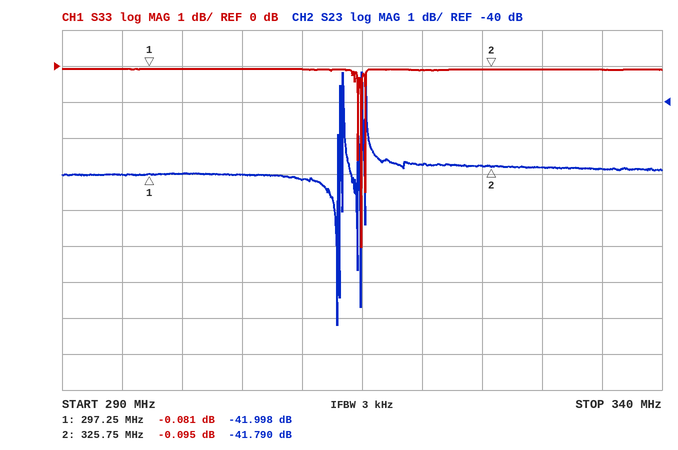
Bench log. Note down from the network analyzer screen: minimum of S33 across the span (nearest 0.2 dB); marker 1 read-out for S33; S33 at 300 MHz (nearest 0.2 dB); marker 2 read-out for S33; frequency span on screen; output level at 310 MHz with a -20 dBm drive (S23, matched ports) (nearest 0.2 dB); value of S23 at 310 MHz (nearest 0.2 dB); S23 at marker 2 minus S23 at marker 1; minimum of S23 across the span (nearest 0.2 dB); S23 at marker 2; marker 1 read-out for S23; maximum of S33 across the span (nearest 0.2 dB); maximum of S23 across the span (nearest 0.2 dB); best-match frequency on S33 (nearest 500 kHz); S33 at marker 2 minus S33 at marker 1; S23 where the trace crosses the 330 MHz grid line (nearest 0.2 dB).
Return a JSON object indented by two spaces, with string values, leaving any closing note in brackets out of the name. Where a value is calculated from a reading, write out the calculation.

{
  "minimum of S33 across the span": "-5.0 dB",
  "marker 1 read-out for S33": "-0.081 dB",
  "S33 at 300 MHz": "0.0 dB",
  "marker 2 read-out for S33": "-0.095 dB",
  "frequency span on screen": "50 MHz",
  "output level at 310 MHz with a -20 dBm drive (S23, matched ports)": "-20 dBm + (-42.2 dB) = -62.2 dBm",
  "value of S23 at 310 MHz": "-42.2 dB",
  "S23 at marker 2 minus S23 at marker 1": "-41.79 − (-41.998) = 0.208 dB",
  "minimum of S23 across the span": "-46.2 dB",
  "S23 at marker 2": "-41.790 dB",
  "marker 1 read-out for S23": "-41.998 dB",
  "maximum of S33 across the span": "0.0 dB",
  "maximum of S23 across the span": "-39.2 dB",
  "best-match frequency on S33": "315.0 MHz",
  "S33 at marker 2 minus S33 at marker 1": "-0.095 − (-0.081) = -0.014 dB",
  "S23 where the trace crosses the 330 MHz grid line": "-41.8 dB"
}
